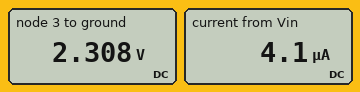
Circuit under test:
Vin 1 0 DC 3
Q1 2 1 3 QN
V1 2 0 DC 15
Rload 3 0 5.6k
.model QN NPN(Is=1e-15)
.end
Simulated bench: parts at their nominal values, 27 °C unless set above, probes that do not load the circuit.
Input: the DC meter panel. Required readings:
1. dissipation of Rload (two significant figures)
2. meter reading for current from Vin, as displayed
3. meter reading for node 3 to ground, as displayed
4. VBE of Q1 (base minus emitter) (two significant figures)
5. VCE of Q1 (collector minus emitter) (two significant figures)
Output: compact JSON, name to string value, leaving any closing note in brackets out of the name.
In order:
{"dissipation of Rload": "950 µW", "meter reading for current from Vin, as displayed": "4.1 µA", "meter reading for node 3 to ground, as displayed": "2.308 V", "VBE of Q1 (base minus emitter)": "690 mV", "VCE of Q1 (collector minus emitter)": "13 V"}
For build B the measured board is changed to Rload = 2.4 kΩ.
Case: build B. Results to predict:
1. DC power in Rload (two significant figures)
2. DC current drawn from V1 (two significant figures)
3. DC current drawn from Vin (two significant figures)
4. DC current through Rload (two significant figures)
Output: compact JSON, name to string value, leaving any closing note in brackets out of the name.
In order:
{"DC power in Rload": "2.2 mW", "DC current drawn from V1": "940 µA", "DC current drawn from Vin": "9.4 µA", "DC current through Rload": "950 µA"}
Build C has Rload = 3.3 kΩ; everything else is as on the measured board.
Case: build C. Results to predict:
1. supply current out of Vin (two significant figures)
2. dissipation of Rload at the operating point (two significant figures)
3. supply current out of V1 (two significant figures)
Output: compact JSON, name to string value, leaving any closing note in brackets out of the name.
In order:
{"supply current out of Vin": "6.9 µA", "dissipation of Rload at the operating point": "1.6 mW", "supply current out of V1": "690 µA"}
